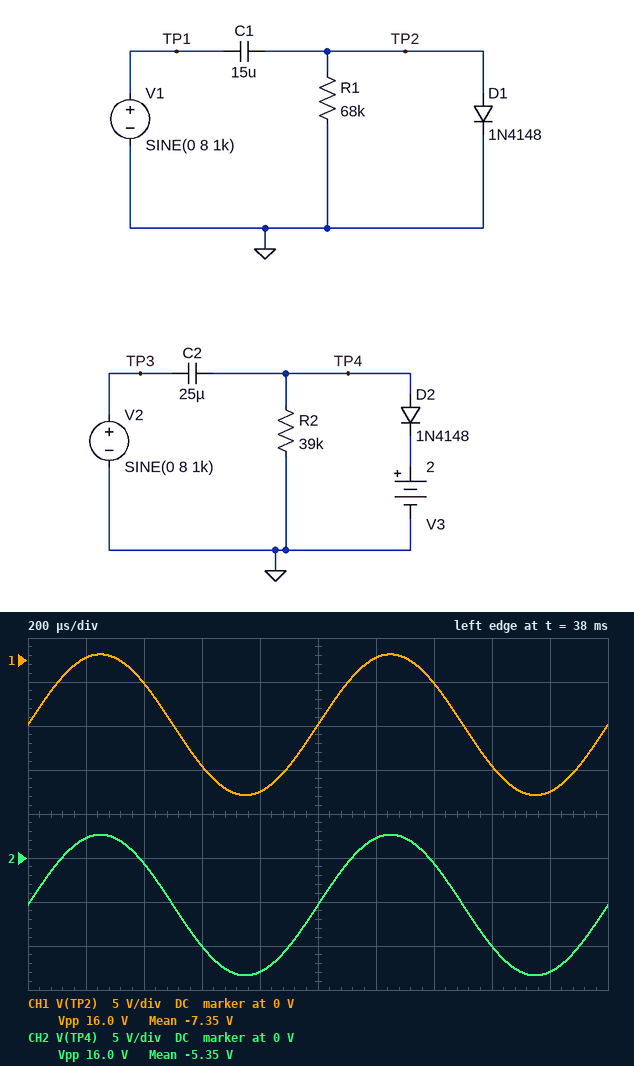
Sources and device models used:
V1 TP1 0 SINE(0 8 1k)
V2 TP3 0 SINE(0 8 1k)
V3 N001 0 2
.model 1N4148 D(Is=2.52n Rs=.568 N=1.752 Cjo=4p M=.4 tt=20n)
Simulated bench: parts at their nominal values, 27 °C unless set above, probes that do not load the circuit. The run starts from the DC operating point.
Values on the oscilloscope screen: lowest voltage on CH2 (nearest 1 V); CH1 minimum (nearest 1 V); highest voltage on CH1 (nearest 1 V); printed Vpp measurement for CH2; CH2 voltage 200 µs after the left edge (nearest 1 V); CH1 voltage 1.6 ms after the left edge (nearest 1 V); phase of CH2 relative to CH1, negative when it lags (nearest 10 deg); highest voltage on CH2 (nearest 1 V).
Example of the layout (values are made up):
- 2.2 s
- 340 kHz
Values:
- -13 V
- -15 V
- 1 V
- 16.0 V
- 2 V
- -12 V
- 0 deg
- 3 V
